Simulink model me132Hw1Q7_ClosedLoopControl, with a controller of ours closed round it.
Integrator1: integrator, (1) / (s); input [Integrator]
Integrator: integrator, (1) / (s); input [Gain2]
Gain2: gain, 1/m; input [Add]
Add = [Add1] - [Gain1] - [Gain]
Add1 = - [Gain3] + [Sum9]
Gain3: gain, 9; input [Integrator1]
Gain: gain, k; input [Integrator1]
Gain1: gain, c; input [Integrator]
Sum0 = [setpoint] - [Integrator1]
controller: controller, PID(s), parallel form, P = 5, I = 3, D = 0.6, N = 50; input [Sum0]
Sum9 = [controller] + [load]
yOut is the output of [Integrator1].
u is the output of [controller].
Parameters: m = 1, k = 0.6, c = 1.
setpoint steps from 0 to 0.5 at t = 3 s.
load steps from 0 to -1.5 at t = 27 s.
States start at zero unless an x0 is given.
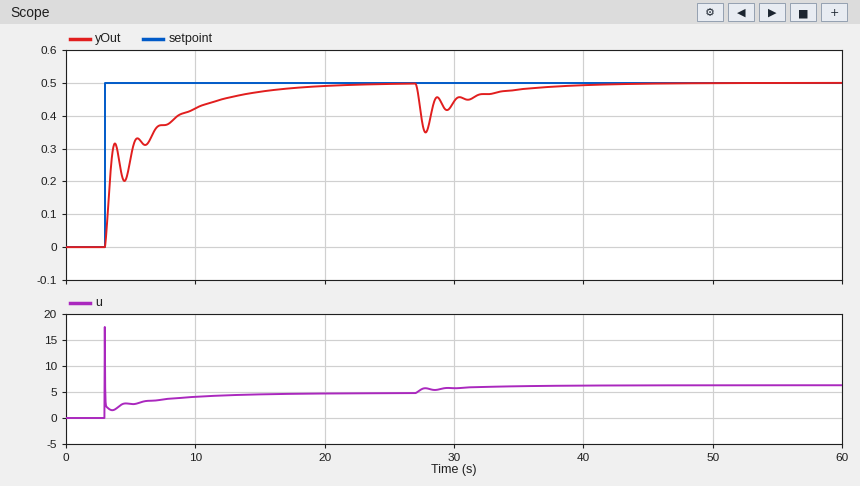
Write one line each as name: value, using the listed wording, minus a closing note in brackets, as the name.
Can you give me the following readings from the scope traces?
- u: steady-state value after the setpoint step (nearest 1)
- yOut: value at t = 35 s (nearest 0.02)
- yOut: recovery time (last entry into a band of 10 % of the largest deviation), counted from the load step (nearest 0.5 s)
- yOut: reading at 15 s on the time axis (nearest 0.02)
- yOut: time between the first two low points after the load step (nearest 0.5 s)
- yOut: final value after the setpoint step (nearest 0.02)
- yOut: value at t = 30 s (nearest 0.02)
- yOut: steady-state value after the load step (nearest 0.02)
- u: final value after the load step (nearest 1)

u: steady-state value after the setpoint step: 5
yOut: value at t = 35 s: 0.48
yOut: recovery time (last entry into a band of 10 % of the largest deviation), counted from the load step: 9.5 s
yOut: reading at 15 s on the time axis: 0.48
yOut: time between the first two low points after the load step: 1.5 s
yOut: final value after the setpoint step: 0.50
yOut: value at t = 30 s: 0.44
yOut: steady-state value after the load step: 0.50
u: final value after the load step: 6
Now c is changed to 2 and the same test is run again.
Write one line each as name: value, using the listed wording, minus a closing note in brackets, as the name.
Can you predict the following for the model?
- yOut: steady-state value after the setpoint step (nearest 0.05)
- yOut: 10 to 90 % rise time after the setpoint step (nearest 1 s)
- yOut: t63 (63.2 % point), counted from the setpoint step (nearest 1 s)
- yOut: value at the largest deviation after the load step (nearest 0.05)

yOut: steady-state value after the setpoint step: 0.50
yOut: 10 to 90 % rise time after the setpoint step: 9 s
yOut: t63 (63.2 % point), counted from the setpoint step: 3 s
yOut: value at the largest deviation after the load step: 0.35
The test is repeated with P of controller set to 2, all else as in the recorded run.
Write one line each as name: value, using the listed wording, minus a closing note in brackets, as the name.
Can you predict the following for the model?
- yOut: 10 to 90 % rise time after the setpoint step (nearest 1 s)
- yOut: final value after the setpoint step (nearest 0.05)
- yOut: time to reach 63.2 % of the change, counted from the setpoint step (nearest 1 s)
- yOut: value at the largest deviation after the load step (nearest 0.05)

yOut: 10 to 90 % rise time after the setpoint step: 8 s
yOut: final value after the setpoint step: 0.50
yOut: time to reach 63.2 % of the change, counted from the setpoint step: 3 s
yOut: value at the largest deviation after the load step: 0.30
